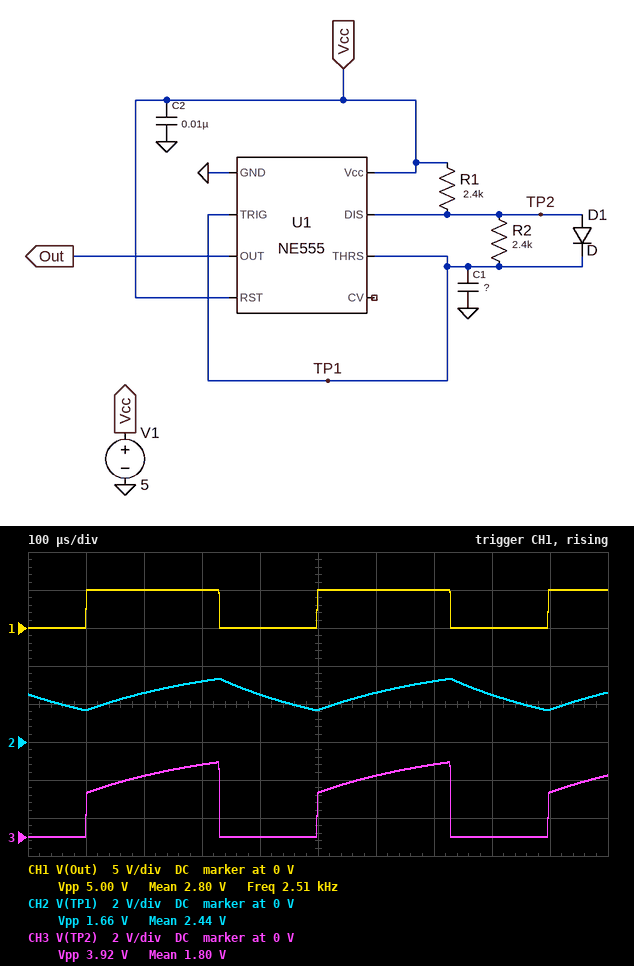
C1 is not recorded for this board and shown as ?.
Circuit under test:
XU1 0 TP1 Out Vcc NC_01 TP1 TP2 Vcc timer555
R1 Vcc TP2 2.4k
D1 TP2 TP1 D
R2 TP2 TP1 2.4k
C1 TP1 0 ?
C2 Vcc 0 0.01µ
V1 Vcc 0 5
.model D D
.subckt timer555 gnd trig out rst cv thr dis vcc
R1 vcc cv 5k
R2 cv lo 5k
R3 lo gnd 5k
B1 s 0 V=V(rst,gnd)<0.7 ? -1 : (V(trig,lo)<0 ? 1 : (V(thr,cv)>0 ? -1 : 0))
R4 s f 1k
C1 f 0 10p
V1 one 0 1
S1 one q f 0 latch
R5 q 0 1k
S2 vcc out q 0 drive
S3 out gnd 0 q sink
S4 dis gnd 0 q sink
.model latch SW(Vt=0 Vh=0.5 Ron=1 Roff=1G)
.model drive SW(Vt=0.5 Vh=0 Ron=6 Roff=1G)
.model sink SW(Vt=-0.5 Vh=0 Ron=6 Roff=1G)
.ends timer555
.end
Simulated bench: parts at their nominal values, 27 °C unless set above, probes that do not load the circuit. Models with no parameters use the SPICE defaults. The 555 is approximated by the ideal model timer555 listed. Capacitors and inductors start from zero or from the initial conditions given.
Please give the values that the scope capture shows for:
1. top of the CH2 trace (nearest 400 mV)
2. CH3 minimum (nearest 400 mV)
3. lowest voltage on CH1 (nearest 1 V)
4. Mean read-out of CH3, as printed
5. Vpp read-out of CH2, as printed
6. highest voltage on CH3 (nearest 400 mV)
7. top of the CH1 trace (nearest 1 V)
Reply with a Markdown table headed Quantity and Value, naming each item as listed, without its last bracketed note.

| Quantity | Value |
|---|---|
| top of the CH2 trace | 3.2 V |
| CH3 minimum | 0 V |
| lowest voltage on CH1 | 0 V |
| Mean read-out of CH3, as printed | 1.80 V |
| Vpp read-out of CH2, as printed | 1.66 V |
| highest voltage on CH3 | 4.0 V |
| top of the CH1 trace | 5 V |
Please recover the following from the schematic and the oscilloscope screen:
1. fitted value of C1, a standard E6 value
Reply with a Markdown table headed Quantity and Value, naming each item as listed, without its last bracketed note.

| Quantity | Value |
|---|---|
| fitted value of C1, a standard E6 value | 100 nF |
